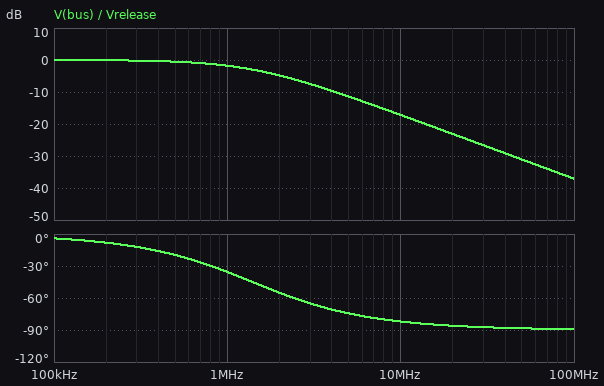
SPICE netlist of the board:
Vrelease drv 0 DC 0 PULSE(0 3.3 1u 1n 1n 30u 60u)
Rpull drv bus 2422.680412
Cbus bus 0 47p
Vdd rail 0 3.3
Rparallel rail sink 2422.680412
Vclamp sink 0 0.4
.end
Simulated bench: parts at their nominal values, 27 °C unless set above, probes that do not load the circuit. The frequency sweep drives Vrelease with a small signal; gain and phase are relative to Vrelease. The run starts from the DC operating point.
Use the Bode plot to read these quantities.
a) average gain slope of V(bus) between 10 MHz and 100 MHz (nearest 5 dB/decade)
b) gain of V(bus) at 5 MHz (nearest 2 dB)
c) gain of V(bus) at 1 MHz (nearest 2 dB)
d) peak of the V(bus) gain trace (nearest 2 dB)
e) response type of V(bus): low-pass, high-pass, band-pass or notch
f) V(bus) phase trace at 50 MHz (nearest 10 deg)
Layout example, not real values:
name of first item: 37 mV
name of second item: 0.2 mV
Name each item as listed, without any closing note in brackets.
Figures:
average gain slope of V(bus) between 10 MHz and 100 MHz: -20 dB/decade
gain of V(bus) at 5 MHz: -12 dB
gain of V(bus) at 1 MHz: -2 dB
peak of the V(bus) gain trace: 0 dB
response type of V(bus): low-pass, high-pass, band-pass or notch: low-pass
V(bus) phase trace at 50 MHz: -90 deg
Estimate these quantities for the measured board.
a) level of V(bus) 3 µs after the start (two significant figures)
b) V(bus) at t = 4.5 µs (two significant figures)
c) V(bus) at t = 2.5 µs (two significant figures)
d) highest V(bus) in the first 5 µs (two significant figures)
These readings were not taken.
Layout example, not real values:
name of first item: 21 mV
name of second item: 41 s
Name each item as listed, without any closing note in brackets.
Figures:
level of V(bus) 3 µs after the start: 3.3 V
V(bus) at t = 4.5 µs: 3.3 V
V(bus) at t = 2.5 µs: 3.3 V
highest V(bus) in the first 5 µs: 3.3 V
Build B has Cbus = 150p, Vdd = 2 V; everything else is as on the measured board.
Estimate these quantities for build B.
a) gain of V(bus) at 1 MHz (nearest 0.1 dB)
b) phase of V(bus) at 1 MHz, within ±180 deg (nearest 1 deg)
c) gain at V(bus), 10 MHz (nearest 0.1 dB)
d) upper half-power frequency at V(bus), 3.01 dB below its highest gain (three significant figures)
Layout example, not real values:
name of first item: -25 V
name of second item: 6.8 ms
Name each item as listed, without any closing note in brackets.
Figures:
gain of V(bus) at 1 MHz: -7.9 dB
phase of V(bus) at 1 MHz, within ±180 deg: -66 deg
gain at V(bus), 10 MHz: -27.2 dB
upper half-power frequency at V(bus), 3.01 dB below its highest gain: 438 kHz
